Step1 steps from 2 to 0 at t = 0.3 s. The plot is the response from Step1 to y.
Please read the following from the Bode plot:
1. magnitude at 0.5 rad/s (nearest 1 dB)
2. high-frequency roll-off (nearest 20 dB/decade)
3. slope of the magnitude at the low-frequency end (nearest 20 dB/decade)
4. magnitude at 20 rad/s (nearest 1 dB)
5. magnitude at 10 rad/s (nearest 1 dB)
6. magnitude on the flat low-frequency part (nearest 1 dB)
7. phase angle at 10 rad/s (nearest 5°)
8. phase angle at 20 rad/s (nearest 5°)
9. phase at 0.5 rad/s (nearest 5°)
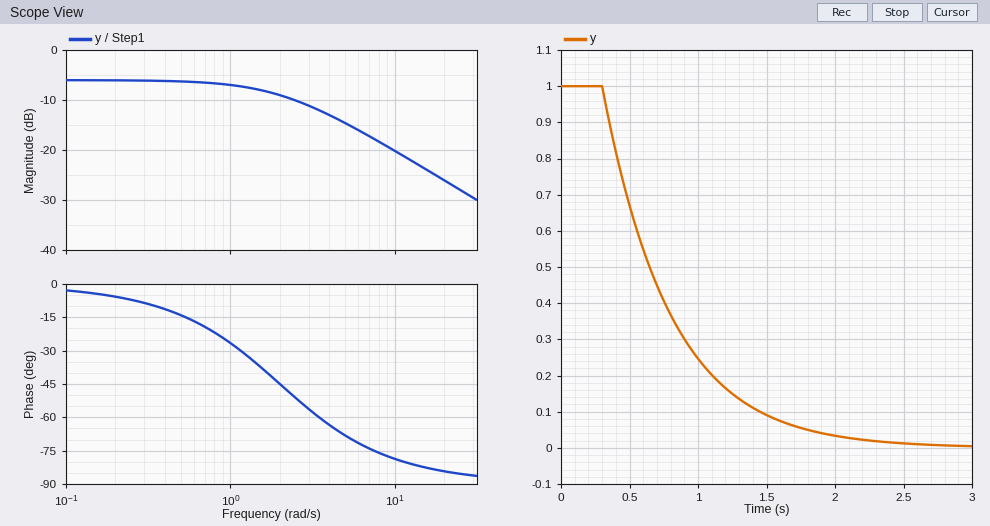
-6 dB
-20 dB/decade
0 dB/decade
-26 dB
-20 dB
-6 dB
-80°
-85°
-15°
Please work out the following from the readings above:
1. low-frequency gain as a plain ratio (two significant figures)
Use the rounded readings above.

0.50
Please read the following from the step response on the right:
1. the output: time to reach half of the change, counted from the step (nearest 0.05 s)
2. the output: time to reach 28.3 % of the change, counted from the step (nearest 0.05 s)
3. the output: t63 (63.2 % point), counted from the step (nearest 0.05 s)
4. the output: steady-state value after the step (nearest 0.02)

0.35 s
0.15 s
0.50 s
0.00
